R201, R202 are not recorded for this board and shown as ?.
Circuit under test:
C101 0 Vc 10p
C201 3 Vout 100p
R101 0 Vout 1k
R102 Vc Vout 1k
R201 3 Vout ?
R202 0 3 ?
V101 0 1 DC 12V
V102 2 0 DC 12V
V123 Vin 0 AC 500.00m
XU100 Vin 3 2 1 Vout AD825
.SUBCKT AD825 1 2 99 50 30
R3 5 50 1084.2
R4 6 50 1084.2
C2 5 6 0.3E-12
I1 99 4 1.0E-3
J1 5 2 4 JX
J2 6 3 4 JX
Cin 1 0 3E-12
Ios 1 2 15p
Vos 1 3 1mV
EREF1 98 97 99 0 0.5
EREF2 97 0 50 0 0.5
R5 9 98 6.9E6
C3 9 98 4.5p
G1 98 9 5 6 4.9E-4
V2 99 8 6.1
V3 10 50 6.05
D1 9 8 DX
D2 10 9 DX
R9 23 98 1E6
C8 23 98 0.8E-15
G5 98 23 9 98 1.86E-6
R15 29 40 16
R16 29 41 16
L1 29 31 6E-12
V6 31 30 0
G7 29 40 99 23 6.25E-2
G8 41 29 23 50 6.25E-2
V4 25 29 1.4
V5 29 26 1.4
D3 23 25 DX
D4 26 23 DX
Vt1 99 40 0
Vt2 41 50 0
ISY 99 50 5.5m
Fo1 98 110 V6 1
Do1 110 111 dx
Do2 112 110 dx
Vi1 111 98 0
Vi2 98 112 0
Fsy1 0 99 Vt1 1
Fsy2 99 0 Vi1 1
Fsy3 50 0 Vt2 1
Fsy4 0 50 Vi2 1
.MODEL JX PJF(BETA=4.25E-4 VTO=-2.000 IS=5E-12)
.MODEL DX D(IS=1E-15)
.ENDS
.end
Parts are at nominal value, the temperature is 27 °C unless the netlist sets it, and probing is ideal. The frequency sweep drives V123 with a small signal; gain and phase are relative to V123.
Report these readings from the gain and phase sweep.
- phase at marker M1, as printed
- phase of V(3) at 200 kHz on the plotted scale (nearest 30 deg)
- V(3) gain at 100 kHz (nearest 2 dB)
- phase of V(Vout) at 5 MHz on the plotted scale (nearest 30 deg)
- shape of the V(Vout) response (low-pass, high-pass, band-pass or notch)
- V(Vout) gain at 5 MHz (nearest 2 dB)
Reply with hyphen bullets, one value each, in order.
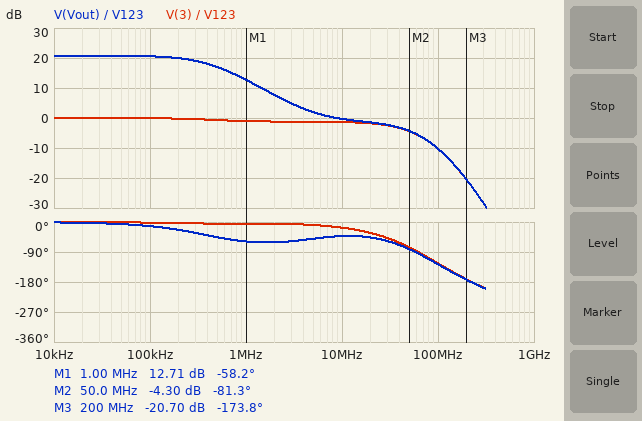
- -58.2 deg
- 0 deg
- 0 dB
- -60 deg
- low-pass
- 2 dB
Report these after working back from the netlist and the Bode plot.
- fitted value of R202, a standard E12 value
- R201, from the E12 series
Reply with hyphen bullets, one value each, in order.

- 330 Ω
- 3.3 kΩ
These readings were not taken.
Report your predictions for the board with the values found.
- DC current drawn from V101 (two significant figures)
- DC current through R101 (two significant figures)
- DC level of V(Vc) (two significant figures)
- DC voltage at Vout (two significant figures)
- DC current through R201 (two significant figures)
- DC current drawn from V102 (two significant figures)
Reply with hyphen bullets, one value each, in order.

- 6.5 mA
- 11 µA
- -11 mV
- -11 mV
- 3.0 µA
- 6.5 mA
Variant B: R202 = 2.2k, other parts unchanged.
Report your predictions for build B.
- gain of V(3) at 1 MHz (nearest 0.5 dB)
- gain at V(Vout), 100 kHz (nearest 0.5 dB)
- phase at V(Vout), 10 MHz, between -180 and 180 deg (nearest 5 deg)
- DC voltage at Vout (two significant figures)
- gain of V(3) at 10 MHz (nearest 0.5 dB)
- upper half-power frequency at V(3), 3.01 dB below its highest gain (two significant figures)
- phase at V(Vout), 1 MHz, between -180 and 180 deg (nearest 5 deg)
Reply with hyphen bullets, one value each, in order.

- 0 dB
- 8.0 dB
- -20 deg
- -2.5 mV
- -0.5 dB
- 44 MHz
- -25 deg
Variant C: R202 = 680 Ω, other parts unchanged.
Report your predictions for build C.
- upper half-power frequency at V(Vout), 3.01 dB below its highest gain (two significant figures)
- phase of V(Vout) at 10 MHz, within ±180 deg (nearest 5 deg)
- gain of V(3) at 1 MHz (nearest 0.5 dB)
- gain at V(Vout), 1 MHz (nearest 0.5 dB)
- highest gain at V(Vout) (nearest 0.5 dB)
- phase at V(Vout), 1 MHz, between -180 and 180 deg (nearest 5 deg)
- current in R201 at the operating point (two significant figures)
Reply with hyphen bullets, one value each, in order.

- 460 kHz
- -30 deg
- -0.5 dB
- 8.0 dB
- 15.5 dB
- -50 deg
- 1.5 µA
